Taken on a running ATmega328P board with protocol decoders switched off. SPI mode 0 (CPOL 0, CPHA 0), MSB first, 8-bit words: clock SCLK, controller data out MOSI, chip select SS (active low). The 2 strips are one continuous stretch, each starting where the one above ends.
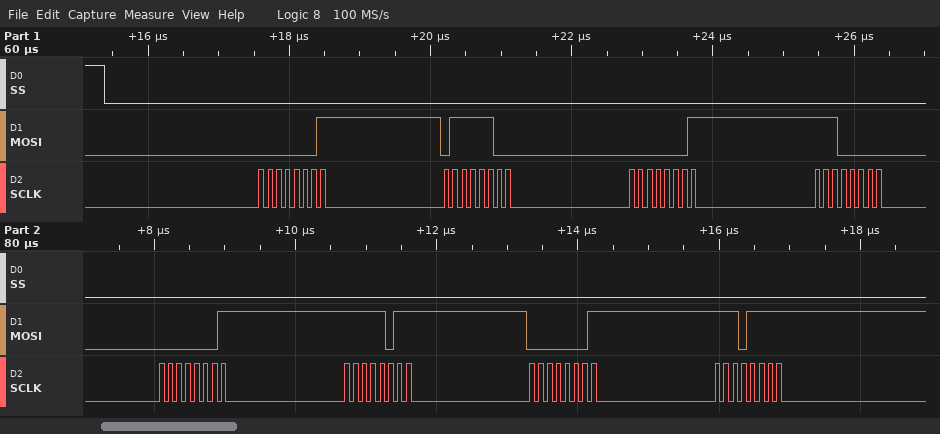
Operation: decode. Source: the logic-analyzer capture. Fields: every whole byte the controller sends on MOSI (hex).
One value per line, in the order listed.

01 7C 01 E0 01 FB 01 EF
